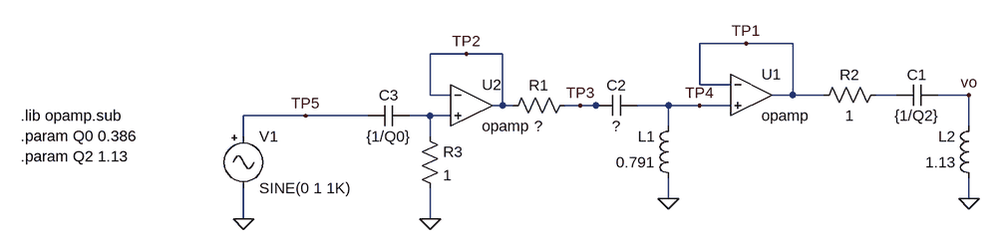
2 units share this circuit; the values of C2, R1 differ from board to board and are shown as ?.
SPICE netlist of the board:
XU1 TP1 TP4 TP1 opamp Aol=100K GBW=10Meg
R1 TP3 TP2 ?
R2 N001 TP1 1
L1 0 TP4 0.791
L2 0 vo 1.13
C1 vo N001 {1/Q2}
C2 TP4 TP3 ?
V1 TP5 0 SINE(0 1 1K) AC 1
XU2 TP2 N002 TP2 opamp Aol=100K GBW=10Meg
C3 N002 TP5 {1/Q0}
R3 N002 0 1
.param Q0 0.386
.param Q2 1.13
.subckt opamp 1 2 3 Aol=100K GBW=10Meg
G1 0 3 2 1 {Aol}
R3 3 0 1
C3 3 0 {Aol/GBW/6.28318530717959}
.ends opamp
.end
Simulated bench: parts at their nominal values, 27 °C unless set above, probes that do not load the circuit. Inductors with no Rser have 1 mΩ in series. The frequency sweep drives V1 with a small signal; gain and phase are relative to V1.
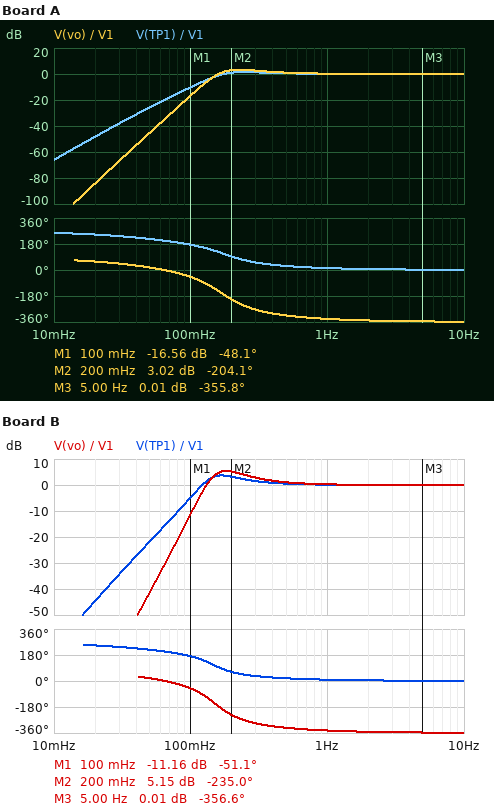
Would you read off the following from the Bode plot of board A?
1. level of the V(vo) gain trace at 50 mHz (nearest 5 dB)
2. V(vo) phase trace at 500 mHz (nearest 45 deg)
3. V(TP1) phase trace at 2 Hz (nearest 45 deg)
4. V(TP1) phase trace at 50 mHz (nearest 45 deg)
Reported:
-45 dB
-315 deg
0 deg
225 deg
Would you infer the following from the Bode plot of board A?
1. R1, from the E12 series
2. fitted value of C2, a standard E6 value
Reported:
0.82 Ω
1 F
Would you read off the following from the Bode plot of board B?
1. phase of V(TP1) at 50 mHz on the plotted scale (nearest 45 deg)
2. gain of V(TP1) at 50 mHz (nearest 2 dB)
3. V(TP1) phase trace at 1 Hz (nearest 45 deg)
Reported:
225 deg
-22 dB
0 deg
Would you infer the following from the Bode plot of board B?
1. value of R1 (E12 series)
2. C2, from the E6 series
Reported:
0.47 Ω
1.5 F
